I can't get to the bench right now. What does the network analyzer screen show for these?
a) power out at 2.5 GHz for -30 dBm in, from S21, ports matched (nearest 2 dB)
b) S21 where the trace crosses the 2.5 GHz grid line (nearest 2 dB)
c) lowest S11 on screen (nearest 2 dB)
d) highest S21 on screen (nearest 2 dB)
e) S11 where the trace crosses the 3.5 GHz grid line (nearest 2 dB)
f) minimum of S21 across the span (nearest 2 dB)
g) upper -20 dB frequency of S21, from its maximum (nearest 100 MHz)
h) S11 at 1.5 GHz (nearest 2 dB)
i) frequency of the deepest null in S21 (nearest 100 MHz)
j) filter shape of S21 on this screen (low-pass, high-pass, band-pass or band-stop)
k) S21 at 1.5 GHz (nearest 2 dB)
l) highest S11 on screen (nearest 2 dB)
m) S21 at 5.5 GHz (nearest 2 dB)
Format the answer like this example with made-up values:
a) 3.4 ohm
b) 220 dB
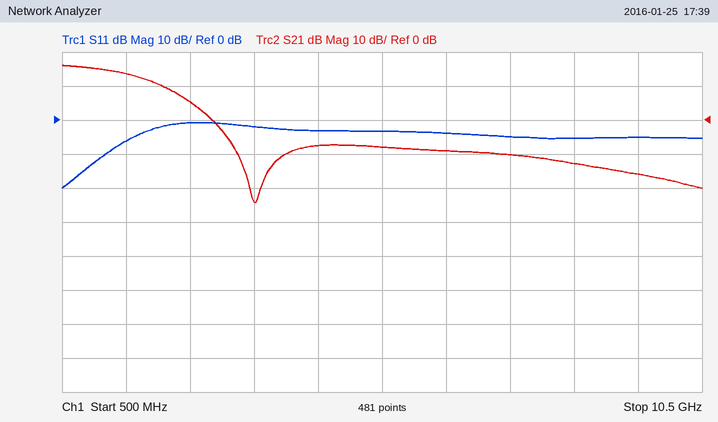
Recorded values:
a) -24 dBm
b) 6 dB
c) -20 dB
d) 16 dB
e) -2 dB
f) -24 dB
g) 3.0 GHz
h) -6 dB
i) 3.5 GHz
j) low-pass
k) 14 dB
l) 0 dB
m) -8 dB
